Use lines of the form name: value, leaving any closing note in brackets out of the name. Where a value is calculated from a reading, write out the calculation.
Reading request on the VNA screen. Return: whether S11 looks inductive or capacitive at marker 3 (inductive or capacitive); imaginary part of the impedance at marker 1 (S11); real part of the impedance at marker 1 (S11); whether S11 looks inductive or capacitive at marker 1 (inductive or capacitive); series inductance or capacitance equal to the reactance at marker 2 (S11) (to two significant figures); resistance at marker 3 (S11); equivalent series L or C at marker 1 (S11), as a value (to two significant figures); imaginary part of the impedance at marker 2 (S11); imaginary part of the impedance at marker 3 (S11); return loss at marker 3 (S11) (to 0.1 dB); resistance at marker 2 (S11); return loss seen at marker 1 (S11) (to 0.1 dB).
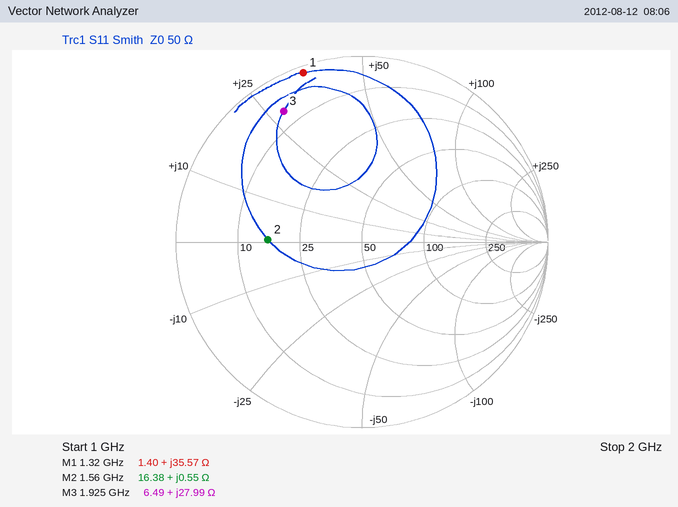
whether S11 looks inductive or capacitive at marker 3: inductive
imaginary part of the impedance at marker 1: +35.57 Ω
real part of the impedance at marker 1: 1.40 Ω
whether S11 looks inductive or capacitive at marker 1: inductive
series inductance or capacitance equal to the reactance at marker 2 (S11): L = 0.55 Ω/(2π × 1.56 GHz) ≈ 56 pH
resistance at marker 3: 6.49 Ω
equivalent series L or C at marker 1 (S11), as a value: L = 35.57 Ω/(2π × 1.32 GHz) ≈ 4.3 nH
imaginary part of the impedance at marker 2: +0.55 Ω
imaginary part of the impedance at marker 3: +27.99 Ω
return loss at marker 3 (S11): 1.7 dB
resistance at marker 2: 16.38 Ω
return loss seen at marker 1 (S11): 0.3 dB
